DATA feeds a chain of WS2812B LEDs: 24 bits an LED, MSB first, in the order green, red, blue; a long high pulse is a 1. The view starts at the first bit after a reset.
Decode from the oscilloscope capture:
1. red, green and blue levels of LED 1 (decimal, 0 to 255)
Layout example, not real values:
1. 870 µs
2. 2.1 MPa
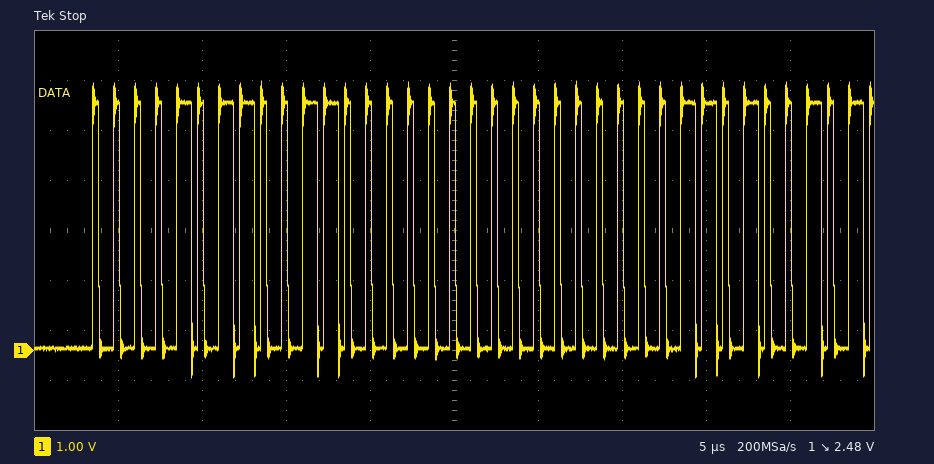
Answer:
1. 48, 11, 0
